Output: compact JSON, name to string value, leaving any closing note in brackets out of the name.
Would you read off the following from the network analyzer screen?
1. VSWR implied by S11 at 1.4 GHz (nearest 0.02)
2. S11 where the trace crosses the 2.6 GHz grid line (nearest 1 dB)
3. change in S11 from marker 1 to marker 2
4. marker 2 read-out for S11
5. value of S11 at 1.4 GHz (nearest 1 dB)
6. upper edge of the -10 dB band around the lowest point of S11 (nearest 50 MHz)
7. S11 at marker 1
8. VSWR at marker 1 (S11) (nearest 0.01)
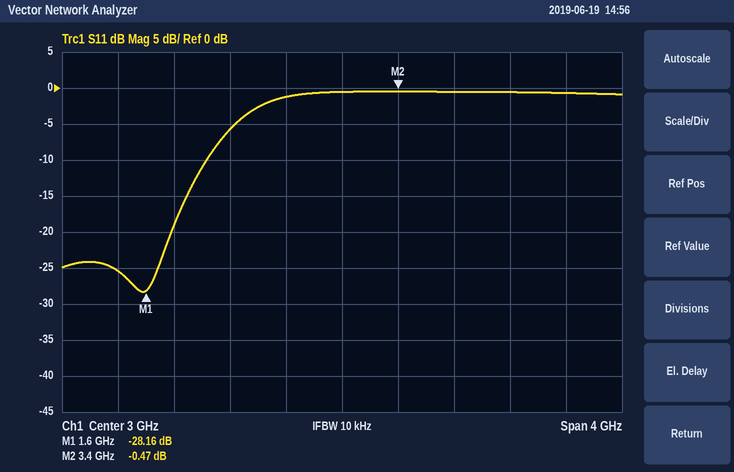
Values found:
{"VSWR implied by S11 at 1.4 GHz": "1.12", "S11 where the trace crosses the 2.6 GHz grid line": "-1 dB", "change in S11 from marker 1 to marker 2": "27.69 dB", "marker 2 read-out for S11": "-0.47 dB", "value of S11 at 1.4 GHz": "-25 dB", "upper edge of the -10 dB band around the lowest point of S11": "2.05 GHz", "S11 at marker 1": "-28.16 dB", "VSWR at marker 1 (S11)": "1.08"}
